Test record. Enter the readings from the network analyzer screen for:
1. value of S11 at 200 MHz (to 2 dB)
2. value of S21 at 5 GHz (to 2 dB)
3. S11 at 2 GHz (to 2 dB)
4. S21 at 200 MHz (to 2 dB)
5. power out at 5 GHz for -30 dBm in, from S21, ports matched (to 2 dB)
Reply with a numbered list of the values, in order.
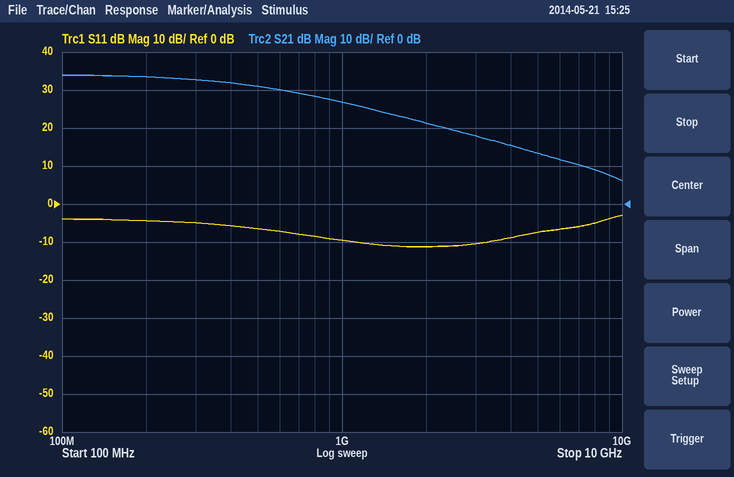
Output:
1. -4 dB
2. 14 dB
3. -12 dB
4. 34 dB
5. -16 dBm
